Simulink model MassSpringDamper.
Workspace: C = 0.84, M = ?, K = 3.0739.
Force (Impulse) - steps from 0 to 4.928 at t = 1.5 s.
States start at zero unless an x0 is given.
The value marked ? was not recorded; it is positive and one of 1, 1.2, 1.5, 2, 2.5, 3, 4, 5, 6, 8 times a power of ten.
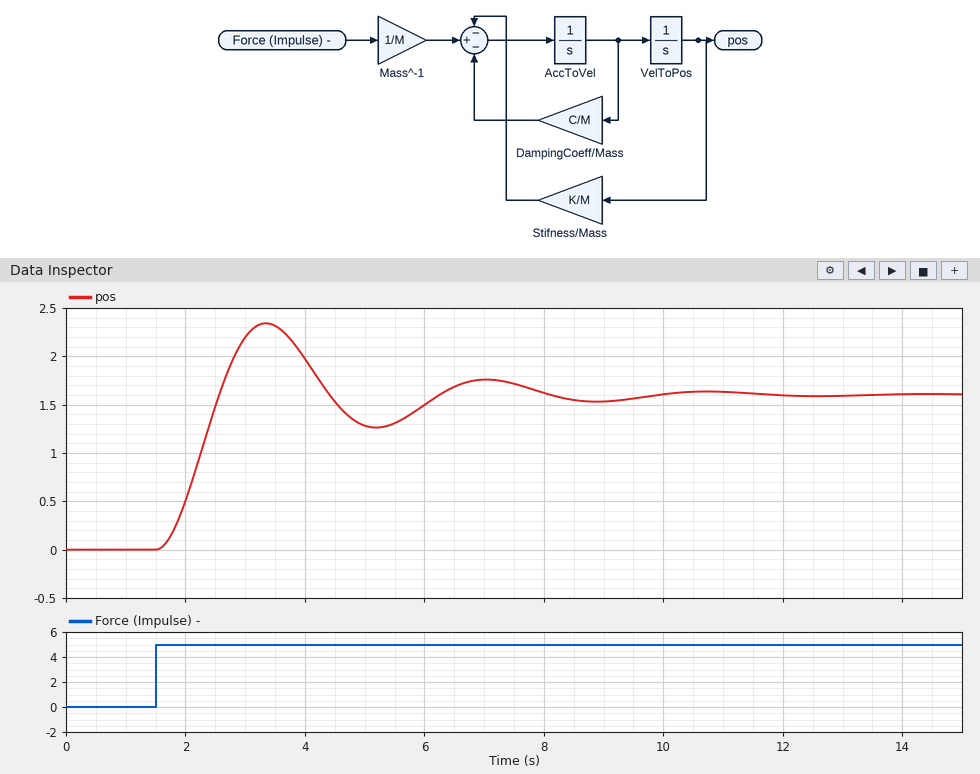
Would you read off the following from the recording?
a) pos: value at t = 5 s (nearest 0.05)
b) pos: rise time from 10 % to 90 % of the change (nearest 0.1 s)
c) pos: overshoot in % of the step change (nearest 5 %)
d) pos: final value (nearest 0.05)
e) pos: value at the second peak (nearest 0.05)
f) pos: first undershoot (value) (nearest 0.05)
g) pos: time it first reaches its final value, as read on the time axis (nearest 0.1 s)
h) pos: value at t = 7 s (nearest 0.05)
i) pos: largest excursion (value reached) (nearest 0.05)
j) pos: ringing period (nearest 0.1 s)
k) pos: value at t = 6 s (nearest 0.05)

1.30
0.7 s
45 %
1.60
1.75
1.25
2.6 s
1.75
2.35
3.7 s
1.50
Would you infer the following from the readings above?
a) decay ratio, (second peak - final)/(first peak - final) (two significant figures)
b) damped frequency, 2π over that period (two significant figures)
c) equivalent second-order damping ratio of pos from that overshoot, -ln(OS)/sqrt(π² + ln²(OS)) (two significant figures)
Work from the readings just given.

0.20
1.7 rad/s
0.25
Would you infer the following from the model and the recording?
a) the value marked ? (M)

1
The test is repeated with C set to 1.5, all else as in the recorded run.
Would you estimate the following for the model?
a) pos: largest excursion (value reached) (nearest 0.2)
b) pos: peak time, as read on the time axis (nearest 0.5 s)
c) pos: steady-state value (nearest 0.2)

2.0
3.5 s
1.6
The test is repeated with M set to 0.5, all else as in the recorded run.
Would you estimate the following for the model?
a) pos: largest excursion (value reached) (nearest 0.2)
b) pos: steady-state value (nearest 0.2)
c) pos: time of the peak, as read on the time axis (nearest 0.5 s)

2.2
1.6
3.0 s
